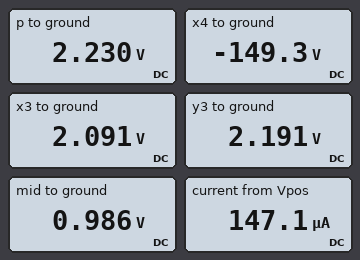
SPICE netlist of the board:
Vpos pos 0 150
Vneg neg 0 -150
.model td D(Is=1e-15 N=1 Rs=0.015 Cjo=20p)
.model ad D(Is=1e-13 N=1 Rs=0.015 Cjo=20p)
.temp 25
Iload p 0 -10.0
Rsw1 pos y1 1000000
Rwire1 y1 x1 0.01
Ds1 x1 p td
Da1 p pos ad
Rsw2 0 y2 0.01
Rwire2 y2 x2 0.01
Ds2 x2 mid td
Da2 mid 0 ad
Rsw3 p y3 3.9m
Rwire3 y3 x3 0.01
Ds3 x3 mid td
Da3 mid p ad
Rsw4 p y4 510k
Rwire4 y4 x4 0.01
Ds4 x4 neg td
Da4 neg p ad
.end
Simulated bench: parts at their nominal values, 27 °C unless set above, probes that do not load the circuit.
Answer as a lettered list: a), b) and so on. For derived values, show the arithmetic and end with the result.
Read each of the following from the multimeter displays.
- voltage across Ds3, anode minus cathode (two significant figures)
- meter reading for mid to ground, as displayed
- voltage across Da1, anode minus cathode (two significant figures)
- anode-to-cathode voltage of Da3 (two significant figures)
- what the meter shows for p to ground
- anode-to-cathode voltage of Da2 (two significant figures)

a) 2.091 V - 986 mV = 1.1 V
b) 0.986 V
c) 2.23 V - 150 V = -150 V
d) 986 mV - 2.23 V = -1.2 V
e) 2.230 V
f) 986 mV = 990 mV
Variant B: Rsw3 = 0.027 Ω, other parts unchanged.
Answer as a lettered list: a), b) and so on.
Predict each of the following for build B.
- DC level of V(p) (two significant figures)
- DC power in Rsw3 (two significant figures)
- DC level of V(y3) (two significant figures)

a) 2.5 V
b) 2.7 W
c) 2.2 V
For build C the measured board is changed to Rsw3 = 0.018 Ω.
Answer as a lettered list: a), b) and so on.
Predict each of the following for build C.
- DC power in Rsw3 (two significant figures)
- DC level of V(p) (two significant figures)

a) 1.8 W
b) 2.4 V
